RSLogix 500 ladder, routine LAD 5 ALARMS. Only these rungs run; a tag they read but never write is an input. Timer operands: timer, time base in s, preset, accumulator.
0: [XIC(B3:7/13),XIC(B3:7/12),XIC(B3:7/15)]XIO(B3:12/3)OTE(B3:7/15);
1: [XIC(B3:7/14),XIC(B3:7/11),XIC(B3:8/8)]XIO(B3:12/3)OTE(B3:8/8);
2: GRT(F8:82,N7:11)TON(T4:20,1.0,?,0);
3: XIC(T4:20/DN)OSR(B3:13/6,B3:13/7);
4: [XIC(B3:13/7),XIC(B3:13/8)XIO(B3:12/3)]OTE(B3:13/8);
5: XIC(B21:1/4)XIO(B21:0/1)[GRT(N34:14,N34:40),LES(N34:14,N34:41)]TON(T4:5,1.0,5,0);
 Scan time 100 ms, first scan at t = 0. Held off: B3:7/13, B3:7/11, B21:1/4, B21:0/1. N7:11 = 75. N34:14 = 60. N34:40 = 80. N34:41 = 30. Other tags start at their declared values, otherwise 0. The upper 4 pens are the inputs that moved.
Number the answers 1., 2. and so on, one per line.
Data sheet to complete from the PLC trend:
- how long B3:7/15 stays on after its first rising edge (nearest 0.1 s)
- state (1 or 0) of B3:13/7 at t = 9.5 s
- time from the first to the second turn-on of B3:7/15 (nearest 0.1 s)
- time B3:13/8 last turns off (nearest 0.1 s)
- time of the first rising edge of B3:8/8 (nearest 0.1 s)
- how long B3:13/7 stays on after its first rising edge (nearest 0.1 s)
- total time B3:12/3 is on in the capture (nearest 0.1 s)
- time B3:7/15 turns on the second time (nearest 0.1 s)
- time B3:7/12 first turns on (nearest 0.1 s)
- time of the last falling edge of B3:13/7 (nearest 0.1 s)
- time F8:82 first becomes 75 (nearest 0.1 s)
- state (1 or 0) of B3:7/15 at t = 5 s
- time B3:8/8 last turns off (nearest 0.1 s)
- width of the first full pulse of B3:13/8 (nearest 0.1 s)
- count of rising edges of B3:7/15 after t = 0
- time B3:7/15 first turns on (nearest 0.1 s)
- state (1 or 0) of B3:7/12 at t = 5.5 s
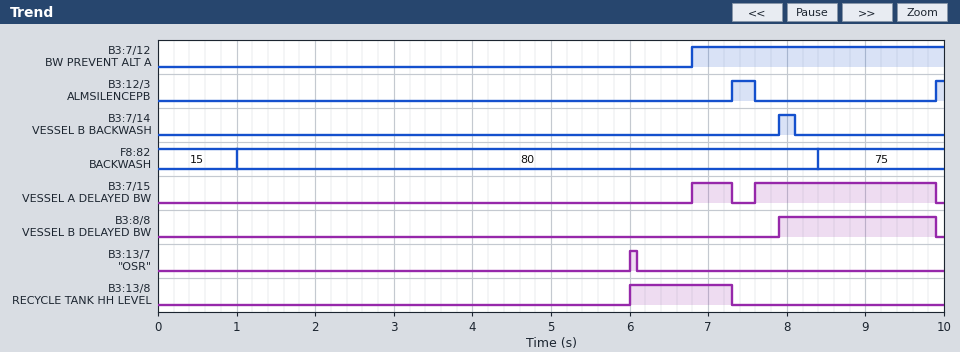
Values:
1. 0.5 s
2. 0
3. 0.8 s
4. 7.3 s
5. 7.9 s
6. 0.1 s
7. 0.4 s
8. 7.6 s
9. 6.8 s
10. 6.1 s
11. 8.4 s
12. 0
13. 9.9 s
14. 1.3 s
15. 2
16. 6.8 s
17. 0
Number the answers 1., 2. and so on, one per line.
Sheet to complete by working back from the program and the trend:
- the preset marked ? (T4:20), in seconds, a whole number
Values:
1. 5 s
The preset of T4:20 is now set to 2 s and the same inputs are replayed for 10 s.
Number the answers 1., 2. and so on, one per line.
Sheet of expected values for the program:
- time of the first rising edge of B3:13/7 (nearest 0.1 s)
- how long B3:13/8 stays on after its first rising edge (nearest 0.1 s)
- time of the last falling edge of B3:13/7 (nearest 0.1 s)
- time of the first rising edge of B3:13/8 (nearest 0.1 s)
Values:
1. 3.0 s
2. 4.3 s
3. 3.1 s
4. 3.0 s
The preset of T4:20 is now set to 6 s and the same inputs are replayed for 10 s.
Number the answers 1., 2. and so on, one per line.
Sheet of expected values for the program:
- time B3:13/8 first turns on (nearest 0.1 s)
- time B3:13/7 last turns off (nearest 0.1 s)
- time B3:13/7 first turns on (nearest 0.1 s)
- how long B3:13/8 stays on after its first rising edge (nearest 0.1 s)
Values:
1. 7.0 s
2. 7.1 s
3. 7.0 s
4. 0.3 s
